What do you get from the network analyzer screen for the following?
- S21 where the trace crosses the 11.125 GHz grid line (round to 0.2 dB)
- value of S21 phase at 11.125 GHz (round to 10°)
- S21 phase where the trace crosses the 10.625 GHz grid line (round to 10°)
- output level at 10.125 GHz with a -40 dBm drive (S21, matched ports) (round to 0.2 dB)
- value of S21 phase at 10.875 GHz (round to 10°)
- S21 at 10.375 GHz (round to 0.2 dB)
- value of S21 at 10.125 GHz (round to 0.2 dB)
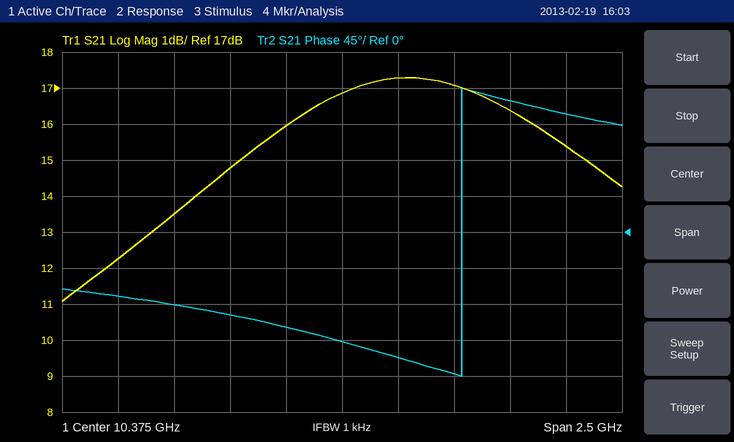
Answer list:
16.4 dB
160°
-160°
-24.0 dBm
-180°
16.8 dB
16.0 dB
